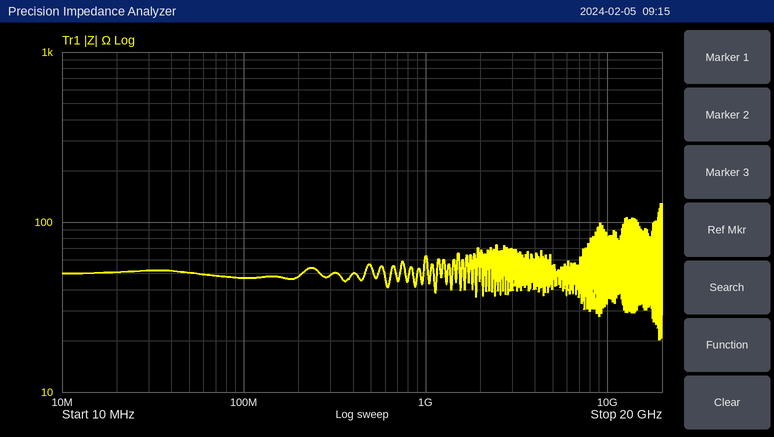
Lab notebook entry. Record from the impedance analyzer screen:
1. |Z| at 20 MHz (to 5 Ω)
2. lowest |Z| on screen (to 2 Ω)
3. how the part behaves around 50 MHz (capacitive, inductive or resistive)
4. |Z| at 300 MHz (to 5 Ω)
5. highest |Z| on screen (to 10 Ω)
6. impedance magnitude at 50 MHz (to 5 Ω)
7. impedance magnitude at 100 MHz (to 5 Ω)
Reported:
50 Ω
20 Ω
resistive
50 Ω
130 Ω
50 Ω
45 Ω
